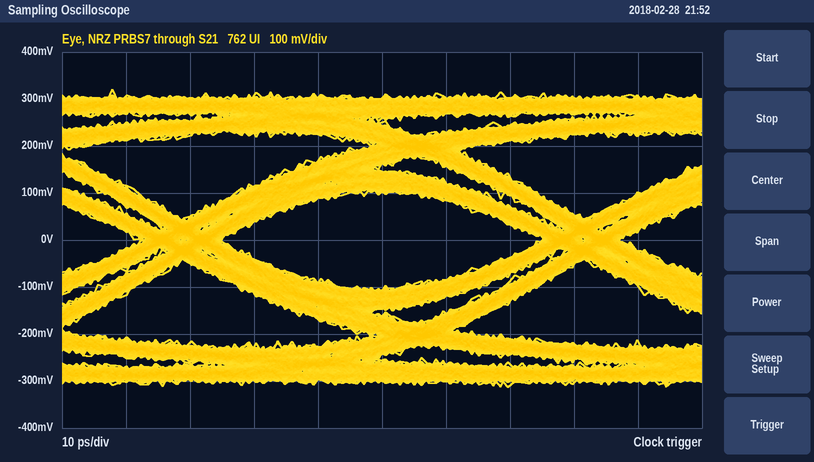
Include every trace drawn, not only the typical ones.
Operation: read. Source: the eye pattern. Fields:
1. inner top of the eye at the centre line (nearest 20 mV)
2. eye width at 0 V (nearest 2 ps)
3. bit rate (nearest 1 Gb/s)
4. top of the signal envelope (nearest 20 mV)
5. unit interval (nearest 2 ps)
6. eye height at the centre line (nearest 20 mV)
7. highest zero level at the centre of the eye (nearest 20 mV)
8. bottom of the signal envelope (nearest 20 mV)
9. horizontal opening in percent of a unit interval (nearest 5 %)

100 mV
50 ps
16 Gb/s
320 mV
62 ps
200 mV
-100 mV
-320 mV
80 %
